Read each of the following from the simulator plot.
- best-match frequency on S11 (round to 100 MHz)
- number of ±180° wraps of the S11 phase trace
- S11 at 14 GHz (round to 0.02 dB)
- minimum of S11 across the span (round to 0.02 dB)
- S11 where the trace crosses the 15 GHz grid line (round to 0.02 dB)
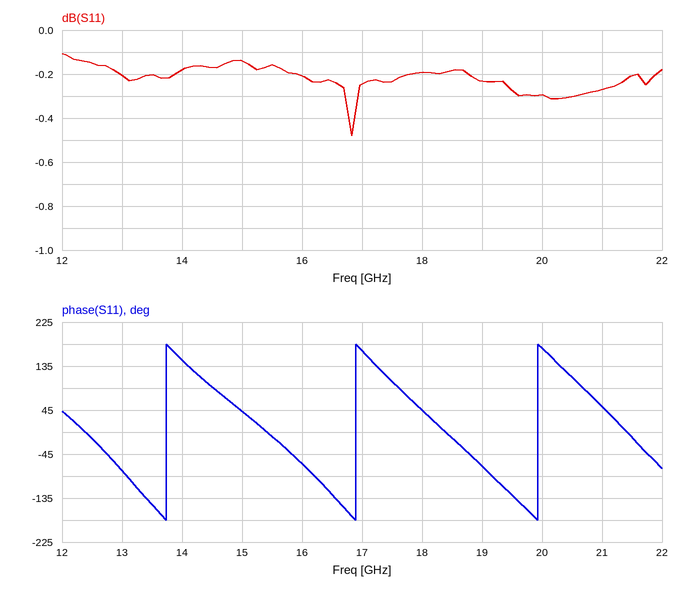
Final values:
16.8 GHz
3
-0.18 dB
-0.48 dB
-0.14 dB
